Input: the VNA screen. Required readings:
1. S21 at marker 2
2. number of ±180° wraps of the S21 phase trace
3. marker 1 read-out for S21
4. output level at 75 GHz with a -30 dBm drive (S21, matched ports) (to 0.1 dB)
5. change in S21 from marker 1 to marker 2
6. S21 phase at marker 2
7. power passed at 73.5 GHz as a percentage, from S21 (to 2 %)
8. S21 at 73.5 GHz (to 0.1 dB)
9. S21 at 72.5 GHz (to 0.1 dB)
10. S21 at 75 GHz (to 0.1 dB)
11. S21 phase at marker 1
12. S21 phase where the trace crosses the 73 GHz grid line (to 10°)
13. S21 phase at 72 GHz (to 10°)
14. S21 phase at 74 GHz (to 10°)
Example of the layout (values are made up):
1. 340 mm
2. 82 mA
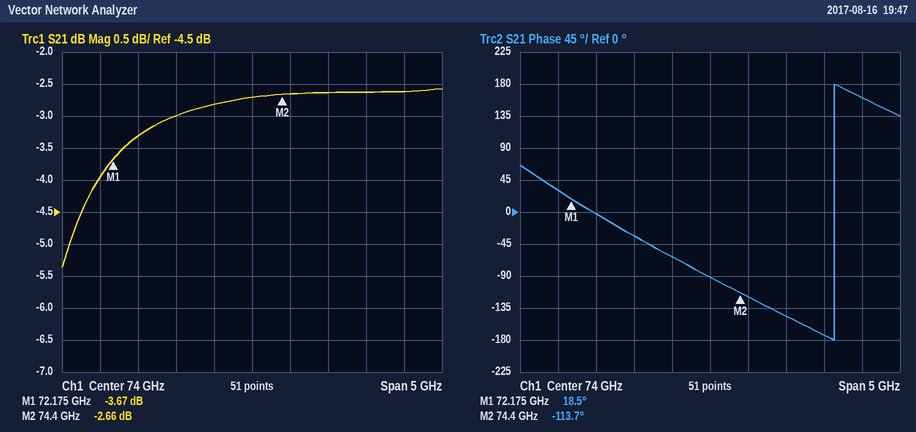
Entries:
1. -2.66 dB
2. 1
3. -3.67 dB
4. -32.6 dBm
5. 1.01 dB
6. -113.7°
7. 52 %
8. -2.8 dB
9. -3.3 dB
10. -2.6 dB
11. 18.5°
12. -30°
13. 30°
14. -90°
